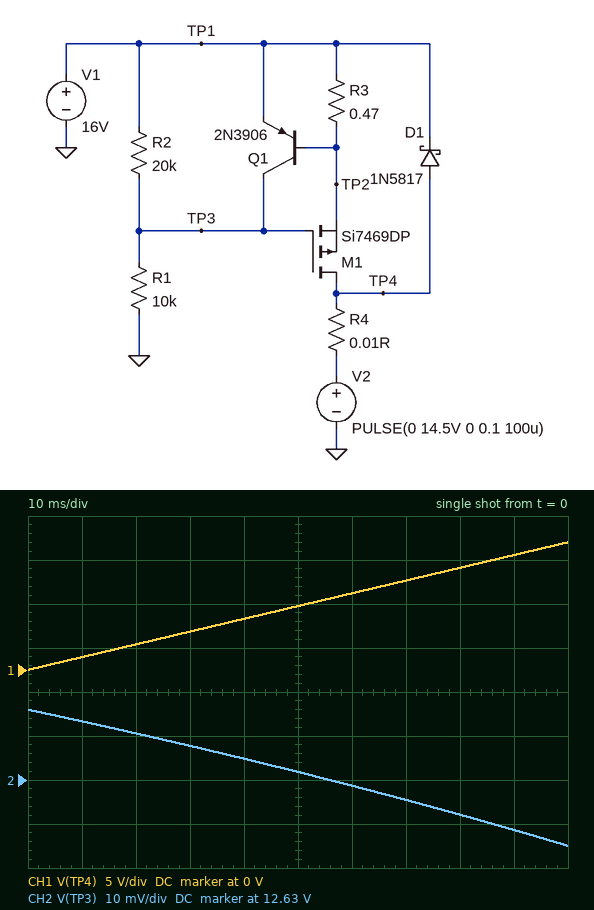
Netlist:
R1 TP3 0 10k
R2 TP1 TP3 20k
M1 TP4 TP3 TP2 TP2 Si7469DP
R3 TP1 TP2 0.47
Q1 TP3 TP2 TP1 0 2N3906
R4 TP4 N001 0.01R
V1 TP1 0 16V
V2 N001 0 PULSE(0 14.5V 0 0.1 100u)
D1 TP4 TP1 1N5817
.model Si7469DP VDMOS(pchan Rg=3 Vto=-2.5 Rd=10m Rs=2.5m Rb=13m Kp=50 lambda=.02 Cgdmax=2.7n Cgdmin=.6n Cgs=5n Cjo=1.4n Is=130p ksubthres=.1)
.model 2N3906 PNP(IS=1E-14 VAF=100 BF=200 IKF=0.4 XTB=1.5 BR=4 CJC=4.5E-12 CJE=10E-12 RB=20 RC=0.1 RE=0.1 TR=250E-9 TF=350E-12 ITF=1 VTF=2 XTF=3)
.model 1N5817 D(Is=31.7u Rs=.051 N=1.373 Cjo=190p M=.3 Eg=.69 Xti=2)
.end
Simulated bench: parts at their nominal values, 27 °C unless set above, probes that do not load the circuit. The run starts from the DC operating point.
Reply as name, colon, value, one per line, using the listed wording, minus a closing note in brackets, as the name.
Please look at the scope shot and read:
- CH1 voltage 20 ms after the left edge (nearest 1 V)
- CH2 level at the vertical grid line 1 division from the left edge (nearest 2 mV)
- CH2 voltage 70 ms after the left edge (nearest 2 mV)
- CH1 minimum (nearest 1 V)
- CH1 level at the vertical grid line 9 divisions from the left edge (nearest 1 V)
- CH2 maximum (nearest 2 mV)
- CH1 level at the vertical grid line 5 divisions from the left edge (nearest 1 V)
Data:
CH1 voltage 20 ms after the left edge: 3 V
CH2 level at the vertical grid line 1 division from the left edge: 12.644 V
CH2 voltage 70 ms after the left edge: 12.626 V
CH1 minimum: 0 V
CH1 level at the vertical grid line 9 divisions from the left edge: 13 V
CH2 maximum: 12.646 V
CH1 level at the vertical grid line 5 divisions from the left edge: 7 V
